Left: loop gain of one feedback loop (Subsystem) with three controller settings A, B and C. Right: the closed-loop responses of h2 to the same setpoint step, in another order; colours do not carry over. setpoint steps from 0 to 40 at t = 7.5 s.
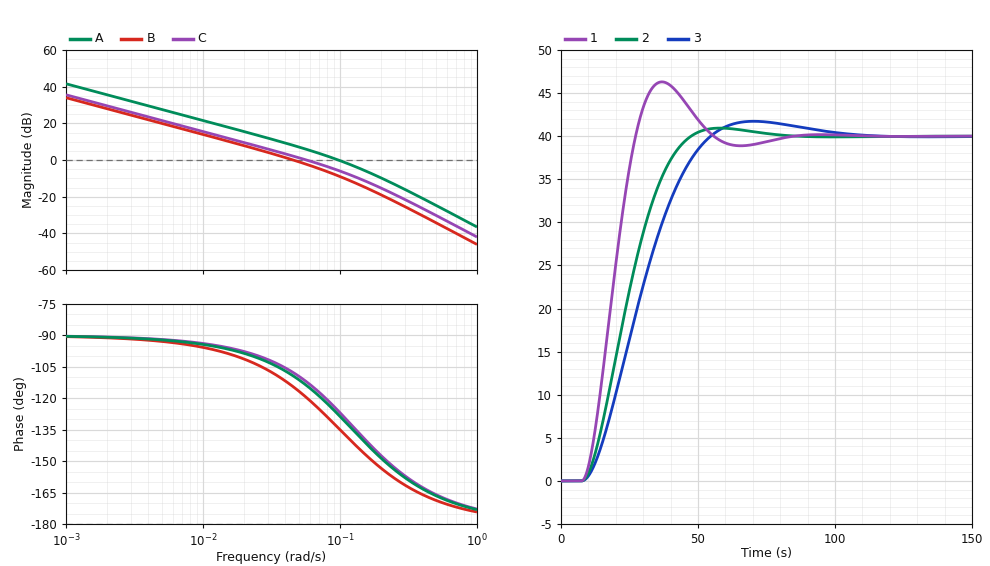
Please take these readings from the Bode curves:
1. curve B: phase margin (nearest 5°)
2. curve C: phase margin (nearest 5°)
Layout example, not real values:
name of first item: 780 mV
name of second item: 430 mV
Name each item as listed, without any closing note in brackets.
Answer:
curve B: phase margin: 65°
curve C: phase margin: 70°
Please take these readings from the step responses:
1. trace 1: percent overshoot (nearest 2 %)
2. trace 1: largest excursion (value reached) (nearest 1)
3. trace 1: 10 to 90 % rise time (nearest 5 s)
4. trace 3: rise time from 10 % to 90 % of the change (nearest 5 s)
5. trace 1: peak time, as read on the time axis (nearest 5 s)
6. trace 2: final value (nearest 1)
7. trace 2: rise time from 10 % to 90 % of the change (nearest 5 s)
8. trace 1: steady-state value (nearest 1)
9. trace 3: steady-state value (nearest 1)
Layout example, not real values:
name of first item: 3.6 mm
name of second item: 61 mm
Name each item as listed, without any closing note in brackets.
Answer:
trace 1: percent overshoot: 16 %
trace 1: largest excursion (value reached): 46
trace 1: 10 to 90 % rise time: 15 s
trace 3: rise time from 10 % to 90 % of the change: 30 s
trace 1: peak time, as read on the time axis: 35 s
trace 2: final value: 40
trace 2: rise time from 10 % to 90 % of the change: 25 s
trace 1: steady-state value: 40
trace 3: steady-state value: 40
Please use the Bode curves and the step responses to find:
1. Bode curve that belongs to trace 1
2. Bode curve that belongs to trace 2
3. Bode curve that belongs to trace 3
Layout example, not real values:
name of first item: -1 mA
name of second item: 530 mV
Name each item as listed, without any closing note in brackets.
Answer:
Bode curve that belongs to trace 1: A
Bode curve that belongs to trace 2: C
Bode curve that belongs to trace 3: B
